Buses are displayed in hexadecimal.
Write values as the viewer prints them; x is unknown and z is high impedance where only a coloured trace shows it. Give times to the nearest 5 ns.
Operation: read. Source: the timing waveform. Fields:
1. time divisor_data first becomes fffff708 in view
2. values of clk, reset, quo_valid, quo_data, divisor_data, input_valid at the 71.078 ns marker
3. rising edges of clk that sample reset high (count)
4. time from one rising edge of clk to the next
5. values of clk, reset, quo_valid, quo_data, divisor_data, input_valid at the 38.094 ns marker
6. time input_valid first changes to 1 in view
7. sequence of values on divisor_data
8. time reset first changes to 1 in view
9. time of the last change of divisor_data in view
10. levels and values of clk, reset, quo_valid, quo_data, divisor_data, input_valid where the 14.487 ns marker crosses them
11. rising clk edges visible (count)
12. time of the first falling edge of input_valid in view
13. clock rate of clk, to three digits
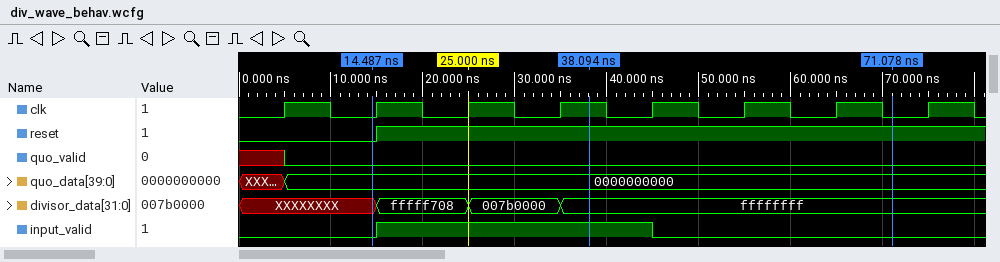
15 ns
clk=0, reset=1, quo_valid=0, quo_data=0000000000, divisor_data=ffffffff, input_valid=0
6
10 ns
clk=1, reset=1, quo_valid=0, quo_data=0000000000, divisor_data=ffffffff, input_valid=1
15 ns
XXXXXXXX, fffff708, 007b0000, ffffffff
15 ns
35 ns
clk=0, reset=0, quo_valid=0, quo_data=0000000000, divisor_data=XXXXXXXX, input_valid=0
8
45 ns
100 MHz
